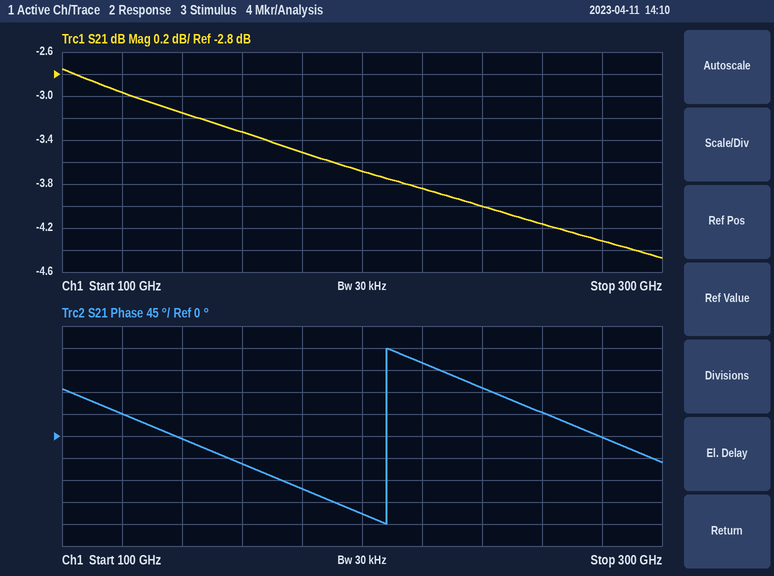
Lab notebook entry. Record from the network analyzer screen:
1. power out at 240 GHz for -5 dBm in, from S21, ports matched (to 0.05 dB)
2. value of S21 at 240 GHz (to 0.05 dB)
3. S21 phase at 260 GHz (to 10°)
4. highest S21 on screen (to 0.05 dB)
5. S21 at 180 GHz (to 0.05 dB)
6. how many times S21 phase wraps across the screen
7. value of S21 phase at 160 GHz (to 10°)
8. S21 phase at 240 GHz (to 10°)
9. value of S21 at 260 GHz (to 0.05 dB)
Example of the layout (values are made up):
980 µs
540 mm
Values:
-9.00 dBm
-4.00 dB
50°
-2.75 dB
-3.50 dB
1
-60°
100°
-4.15 dB
